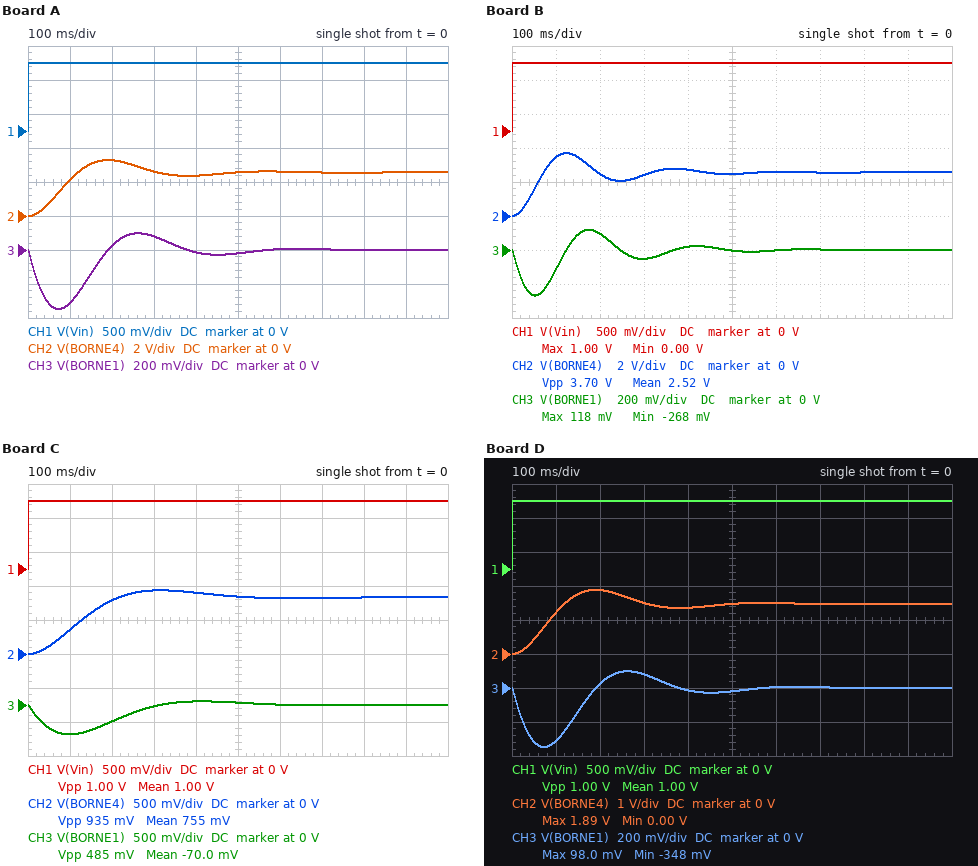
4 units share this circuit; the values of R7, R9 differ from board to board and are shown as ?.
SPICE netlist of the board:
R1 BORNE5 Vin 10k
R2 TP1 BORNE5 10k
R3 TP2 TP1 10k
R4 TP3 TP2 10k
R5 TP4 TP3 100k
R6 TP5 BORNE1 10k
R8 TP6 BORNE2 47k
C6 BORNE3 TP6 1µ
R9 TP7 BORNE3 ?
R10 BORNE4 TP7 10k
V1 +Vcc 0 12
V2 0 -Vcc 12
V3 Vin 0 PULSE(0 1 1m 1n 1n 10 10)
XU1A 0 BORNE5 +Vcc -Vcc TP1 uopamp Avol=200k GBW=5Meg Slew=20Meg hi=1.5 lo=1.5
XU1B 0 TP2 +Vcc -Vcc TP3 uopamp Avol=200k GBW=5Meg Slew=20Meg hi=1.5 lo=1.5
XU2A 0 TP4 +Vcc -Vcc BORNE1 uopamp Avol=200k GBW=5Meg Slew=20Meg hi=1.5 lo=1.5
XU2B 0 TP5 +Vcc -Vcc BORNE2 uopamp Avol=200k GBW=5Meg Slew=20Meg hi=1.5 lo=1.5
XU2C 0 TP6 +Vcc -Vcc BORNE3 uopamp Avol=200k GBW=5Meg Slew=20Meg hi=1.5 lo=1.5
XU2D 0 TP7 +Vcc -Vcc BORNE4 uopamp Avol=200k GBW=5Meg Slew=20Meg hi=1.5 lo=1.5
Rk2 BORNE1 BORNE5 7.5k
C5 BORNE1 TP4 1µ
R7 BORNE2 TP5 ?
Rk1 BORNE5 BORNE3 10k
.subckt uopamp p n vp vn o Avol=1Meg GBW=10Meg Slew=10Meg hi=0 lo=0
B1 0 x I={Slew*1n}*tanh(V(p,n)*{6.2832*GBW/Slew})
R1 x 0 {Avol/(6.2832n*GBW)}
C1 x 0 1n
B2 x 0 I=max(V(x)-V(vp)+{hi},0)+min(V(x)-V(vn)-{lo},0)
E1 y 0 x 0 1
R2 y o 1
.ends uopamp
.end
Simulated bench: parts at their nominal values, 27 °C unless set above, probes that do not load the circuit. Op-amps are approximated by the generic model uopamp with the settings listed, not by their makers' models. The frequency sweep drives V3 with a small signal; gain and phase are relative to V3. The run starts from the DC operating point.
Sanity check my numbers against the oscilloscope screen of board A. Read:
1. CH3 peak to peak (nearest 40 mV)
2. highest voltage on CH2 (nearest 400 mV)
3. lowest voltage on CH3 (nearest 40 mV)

440 mV
3.2 V
-360 mV
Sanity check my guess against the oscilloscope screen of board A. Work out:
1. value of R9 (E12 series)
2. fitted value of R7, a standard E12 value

3.9 kΩ
15 kΩ
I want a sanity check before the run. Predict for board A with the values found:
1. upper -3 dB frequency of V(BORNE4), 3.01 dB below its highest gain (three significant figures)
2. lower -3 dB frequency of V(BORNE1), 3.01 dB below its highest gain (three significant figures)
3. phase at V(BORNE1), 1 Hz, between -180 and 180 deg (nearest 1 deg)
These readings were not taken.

3.38 Hz
1.97 Hz
-107 deg
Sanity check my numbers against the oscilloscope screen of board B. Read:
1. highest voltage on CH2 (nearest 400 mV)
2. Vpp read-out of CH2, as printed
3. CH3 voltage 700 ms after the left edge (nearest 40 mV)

3.6 V
3.70 V
0 V
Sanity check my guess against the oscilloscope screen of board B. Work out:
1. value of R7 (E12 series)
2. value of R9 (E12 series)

33 kΩ
3.9 kΩ
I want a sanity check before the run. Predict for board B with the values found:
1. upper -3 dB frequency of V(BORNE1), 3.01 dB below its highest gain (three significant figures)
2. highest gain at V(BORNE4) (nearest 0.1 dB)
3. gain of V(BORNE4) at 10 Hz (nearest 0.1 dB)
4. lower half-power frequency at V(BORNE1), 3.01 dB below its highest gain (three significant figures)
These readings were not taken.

5.41 Hz
14.4 dB
-5.4 dB
3.29 Hz
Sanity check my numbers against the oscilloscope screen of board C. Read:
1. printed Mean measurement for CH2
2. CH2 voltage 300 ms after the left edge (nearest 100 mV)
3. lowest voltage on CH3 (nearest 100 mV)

755 mV
900 mV
-400 mV
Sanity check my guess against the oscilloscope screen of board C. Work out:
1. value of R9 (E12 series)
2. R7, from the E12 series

12 kΩ
6.8 kΩ
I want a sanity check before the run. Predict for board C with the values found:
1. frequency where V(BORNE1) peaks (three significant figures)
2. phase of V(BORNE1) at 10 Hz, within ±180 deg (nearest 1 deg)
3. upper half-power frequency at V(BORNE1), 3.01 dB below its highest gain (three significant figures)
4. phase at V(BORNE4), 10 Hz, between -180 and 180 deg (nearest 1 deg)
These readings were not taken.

1.91 Hz
102 deg
3.25 Hz
-168 deg
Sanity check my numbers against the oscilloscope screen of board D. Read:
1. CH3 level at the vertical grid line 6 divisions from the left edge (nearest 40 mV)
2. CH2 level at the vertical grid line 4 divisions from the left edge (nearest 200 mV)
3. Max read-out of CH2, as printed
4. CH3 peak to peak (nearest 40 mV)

0 V
1.4 V
1.89 V
440 mV
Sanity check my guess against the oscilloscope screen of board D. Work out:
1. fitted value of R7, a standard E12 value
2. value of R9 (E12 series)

15 kΩ
6.8 kΩ
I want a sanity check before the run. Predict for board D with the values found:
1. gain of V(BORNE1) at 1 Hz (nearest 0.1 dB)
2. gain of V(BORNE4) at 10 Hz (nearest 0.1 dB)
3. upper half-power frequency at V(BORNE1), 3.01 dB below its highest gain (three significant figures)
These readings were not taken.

-13.3 dB
-18.0 dB
4.10 Hz
